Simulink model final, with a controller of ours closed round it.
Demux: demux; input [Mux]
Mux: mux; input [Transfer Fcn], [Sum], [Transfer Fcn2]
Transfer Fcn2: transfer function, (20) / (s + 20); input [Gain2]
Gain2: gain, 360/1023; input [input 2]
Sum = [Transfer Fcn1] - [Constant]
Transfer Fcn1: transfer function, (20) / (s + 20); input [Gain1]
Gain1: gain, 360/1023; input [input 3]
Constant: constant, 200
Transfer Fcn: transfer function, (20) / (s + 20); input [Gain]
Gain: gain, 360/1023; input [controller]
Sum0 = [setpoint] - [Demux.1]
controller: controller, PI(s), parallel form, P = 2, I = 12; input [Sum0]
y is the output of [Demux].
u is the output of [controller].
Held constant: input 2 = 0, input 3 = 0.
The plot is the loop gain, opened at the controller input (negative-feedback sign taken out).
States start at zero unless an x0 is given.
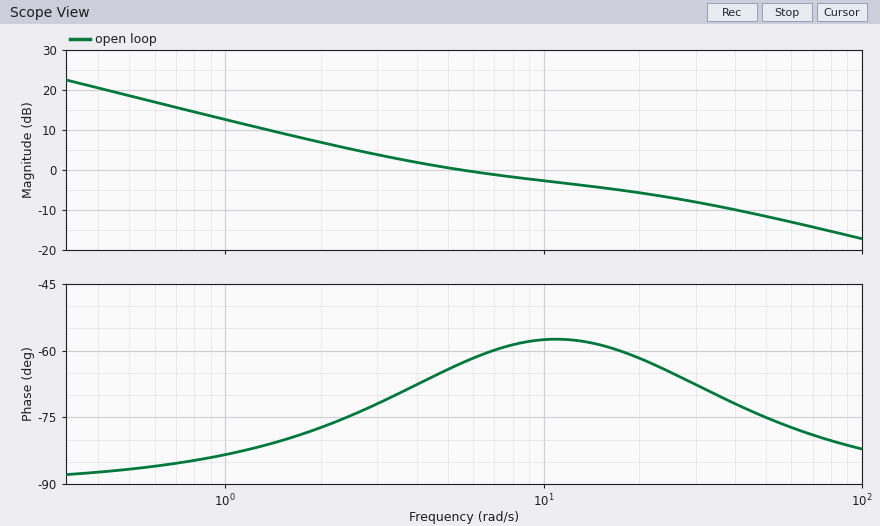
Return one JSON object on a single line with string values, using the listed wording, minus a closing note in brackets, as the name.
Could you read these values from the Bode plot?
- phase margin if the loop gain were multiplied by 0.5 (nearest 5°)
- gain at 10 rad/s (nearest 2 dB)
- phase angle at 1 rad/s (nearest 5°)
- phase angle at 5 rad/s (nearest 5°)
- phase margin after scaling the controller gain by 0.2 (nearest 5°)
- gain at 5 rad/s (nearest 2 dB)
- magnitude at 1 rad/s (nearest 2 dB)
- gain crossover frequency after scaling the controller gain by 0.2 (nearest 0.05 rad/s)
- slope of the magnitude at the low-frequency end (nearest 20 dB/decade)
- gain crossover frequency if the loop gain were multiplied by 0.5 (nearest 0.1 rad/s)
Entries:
{"phase margin if the loop gain were multiplied by 0.5": "105°", "gain at 10 rad/s": "-2 dB", "phase angle at 1 rad/s": "-85°", "phase angle at 5 rad/s": "-65°", "phase margin after scaling the controller gain by 0.2": "95°", "gain at 5 rad/s": "0 dB", "magnitude at 1 rad/s": "12 dB", "gain crossover frequency after scaling the controller gain by 0.2": "0.85 rad/s", "slope of the magnitude at the low-frequency end": "-20 dB/decade", "gain crossover frequency if the loop gain were multiplied by 0.5": "2.2 rad/s"}
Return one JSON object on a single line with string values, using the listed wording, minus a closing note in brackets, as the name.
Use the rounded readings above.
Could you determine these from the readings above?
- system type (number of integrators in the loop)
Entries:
{"system type": "1"}
